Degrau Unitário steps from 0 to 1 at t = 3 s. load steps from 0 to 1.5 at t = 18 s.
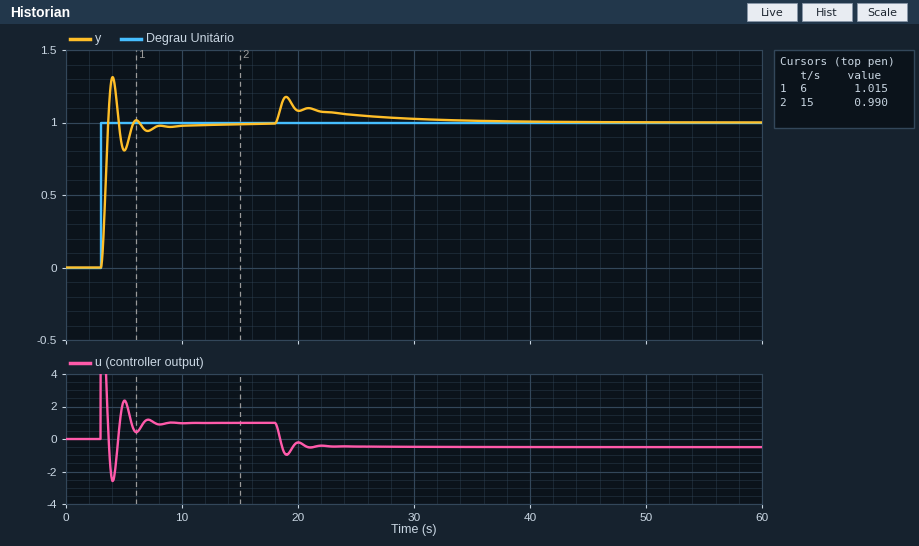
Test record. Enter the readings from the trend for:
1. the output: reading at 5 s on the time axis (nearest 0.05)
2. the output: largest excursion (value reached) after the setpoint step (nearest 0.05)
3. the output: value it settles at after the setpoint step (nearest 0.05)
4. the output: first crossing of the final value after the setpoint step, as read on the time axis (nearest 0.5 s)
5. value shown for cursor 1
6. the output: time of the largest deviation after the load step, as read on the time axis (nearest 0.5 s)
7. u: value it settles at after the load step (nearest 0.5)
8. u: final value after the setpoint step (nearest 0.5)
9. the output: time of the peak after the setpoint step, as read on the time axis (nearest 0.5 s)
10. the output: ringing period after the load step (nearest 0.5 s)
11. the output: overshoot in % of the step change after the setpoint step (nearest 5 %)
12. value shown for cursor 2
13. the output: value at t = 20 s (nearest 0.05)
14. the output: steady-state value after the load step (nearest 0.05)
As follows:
0.80
1.30
1.00
3.5 s
1.015
19.0 s
-0.5
1.0
4.0 s
2.0 s
30 %
0.990
1.10
1.00
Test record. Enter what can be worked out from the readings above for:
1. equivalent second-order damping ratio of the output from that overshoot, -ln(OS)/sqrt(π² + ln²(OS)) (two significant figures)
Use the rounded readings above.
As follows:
0.36
